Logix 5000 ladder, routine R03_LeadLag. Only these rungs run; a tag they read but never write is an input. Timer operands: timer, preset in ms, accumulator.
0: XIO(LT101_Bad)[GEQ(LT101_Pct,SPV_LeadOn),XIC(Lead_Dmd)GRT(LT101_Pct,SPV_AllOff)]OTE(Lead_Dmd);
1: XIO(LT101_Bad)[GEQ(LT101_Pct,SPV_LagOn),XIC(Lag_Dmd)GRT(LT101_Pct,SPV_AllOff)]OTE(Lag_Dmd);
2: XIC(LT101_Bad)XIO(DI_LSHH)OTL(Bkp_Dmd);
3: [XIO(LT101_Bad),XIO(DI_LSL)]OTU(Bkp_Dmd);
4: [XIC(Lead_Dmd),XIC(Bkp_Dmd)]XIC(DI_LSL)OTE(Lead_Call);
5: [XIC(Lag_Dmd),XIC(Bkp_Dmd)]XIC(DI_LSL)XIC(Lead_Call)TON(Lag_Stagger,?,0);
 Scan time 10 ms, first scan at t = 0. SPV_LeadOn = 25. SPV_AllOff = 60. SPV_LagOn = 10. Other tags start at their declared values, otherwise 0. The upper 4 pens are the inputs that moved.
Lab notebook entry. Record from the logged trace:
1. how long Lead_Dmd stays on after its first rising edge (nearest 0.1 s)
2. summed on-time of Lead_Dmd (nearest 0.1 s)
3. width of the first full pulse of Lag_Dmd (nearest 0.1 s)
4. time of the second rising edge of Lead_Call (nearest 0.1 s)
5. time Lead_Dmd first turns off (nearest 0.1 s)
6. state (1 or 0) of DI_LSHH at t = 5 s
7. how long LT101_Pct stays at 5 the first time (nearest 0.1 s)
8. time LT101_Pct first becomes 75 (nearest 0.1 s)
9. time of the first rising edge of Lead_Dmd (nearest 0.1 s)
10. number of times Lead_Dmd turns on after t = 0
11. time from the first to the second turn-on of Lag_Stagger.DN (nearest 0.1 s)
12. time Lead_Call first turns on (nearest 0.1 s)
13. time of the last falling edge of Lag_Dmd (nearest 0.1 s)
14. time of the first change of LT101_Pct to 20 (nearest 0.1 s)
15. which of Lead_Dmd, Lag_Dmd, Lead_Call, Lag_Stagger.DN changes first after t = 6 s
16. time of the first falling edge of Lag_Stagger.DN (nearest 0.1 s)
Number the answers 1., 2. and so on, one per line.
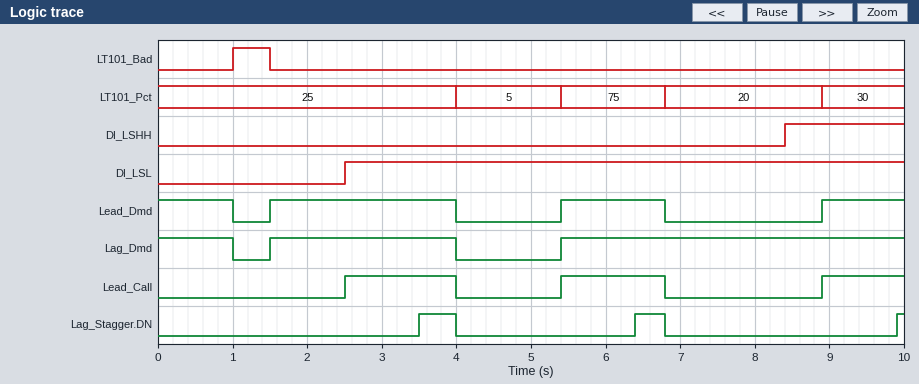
1. 2.5 s
2. 6.0 s
3. 2.5 s
4. 5.4 s
5. 1.0 s
6. 0
7. 1.4 s
8. 5.4 s
9. 1.5 s
10. 3
11. 2.9 s
12. 2.5 s
13. 4.0 s
14. 6.8 s
15. Lag_Stagger.DN
16. 4.0 s
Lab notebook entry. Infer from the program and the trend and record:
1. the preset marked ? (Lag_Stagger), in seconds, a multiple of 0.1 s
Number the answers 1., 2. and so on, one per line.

1. 1.0 s
